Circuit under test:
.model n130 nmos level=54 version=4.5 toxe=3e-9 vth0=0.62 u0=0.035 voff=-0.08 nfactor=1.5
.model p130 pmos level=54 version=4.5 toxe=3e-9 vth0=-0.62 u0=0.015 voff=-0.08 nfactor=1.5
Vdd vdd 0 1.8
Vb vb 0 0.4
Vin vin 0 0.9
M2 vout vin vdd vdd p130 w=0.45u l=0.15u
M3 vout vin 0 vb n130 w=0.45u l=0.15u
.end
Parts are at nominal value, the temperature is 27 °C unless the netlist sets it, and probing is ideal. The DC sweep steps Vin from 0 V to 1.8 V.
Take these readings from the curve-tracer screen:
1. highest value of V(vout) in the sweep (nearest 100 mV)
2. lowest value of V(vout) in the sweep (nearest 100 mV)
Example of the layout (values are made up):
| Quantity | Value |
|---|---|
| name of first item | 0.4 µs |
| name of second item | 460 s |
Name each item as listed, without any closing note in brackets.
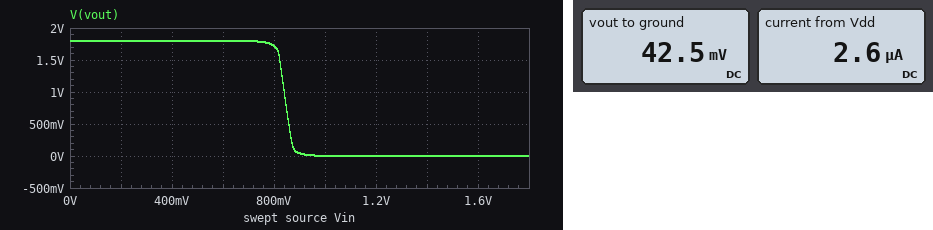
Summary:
| Quantity | Value |
|---|---|
| highest value of V(vout) in the sweep | 1.8 V |
| lowest value of V(vout) in the sweep | 0 V |
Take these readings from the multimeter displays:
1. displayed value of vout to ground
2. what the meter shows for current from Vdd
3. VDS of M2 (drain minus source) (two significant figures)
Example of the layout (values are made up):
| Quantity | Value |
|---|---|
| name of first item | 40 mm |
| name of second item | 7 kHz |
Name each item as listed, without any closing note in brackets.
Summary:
| Quantity | Value |
|---|---|
| displayed value of vout to ground | 42.5 mV |
| what the meter shows for current from Vdd | 2.6 µA |
| VDS of M2 (drain minus source) | -1.8 V |
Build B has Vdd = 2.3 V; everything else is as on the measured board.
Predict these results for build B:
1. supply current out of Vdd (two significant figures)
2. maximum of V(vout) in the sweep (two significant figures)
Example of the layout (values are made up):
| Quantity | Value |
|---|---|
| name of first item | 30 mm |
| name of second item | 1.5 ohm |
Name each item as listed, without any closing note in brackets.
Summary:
| Quantity | Value |
|---|---|
| supply current out of Vdd | 16 µA |
| maximum of V(vout) in the sweep | 2.3 V |
